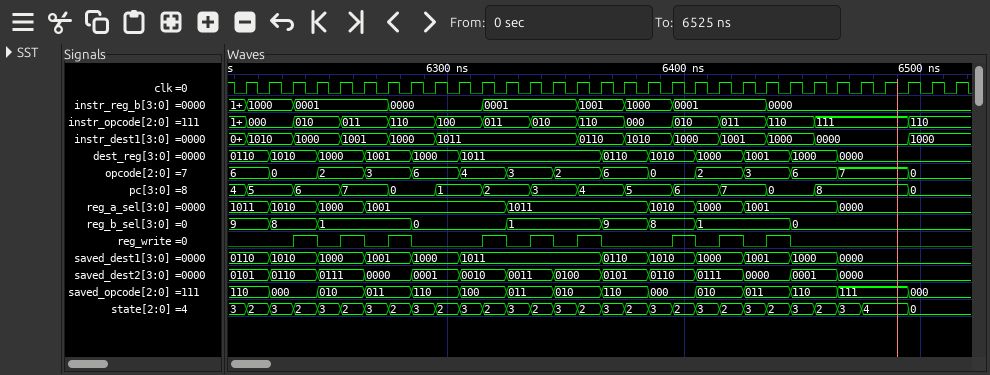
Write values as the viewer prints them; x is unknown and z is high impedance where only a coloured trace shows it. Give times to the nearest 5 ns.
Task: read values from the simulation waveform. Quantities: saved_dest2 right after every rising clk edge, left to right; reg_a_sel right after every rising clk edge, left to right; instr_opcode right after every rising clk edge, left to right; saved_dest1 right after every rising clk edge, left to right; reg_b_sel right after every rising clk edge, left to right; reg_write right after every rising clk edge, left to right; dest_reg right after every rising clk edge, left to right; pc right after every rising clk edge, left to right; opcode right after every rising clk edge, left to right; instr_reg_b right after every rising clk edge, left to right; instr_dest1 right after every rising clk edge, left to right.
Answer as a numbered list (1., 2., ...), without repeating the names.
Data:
1. 0101, 0110, 0110, 0111, 0111, 0000, 0000, 0001, 0001, 0010, 0010, 0011, 0011, 0100, 0100, 0101, 0101, 0110, 0110, 0111, 0111, 0000, 0000, 0001, 0001, 0000, 0000, 0000, 0000, 0000, 0000
2. 1011, 1010, 1010, 1000, 1000, 1001, 1001, 1001, 1001, 1001, 1001, 1011, 1011, 1011, 1011, 1011, 1011, 1010, 1010, 1000, 1000, 1001, 1001, 1001, 1001, 0000, 0000, 0000, 0000, 0000, 0000
3. 000, 000, 010, 010, 011, 011, 110, 110, 100, 100, 011, 011, 010, 010, 110, 110, 000, 000, 010, 010, 011, 011, 110, 110, 111, 111, 111, 111, 110, 110, 110
4. 0110, 1010, 1010, 1000, 1000, 1001, 1001, 1000, 1000, 1011, 1011, 1011, 1011, 1011, 1011, 0110, 0110, 1010, 1010, 1000, 1000, 1001, 1001, 1000, 1000, 0000, 0000, 0000, 0000, 0000, 0000
5. 9, 8, 8, 1, 1, 1, 1, 0, 0, 0, 0, 1, 1, 1, 1, 9, 9, 8, 8, 1, 1, 1, 1, 0, 0, 0, 0, 0, 0, 0, 0
6. 0 0 1 0 1 0 1 0 0 0 1 0 1 0 1 0 0 0 1 0 1 0 1 0 0 0 0 0 0 0 0
7. 0110, 1010, 1010, 1000, 1000, 1001, 1001, 1000, 1000, 1011, 1011, 1011, 1011, 1011, 1011, 0110, 0110, 1010, 1010, 1000, 1000, 1001, 1001, 1000, 1000, 0000, 0000, 0000, 0000, 0000, 0000
8. 5, 5, 6, 6, 7, 7, 0, 0, 1, 1, 2, 2, 3, 3, 4, 4, 5, 5, 6, 6, 7, 7, 0, 0, 8, 8, 8, 8, 0, 0, 0
9. 6, 0, 0, 2, 2, 3, 3, 6, 6, 4, 4, 3, 3, 2, 2, 6, 6, 0, 0, 2, 2, 3, 3, 6, 6, 7, 7, 7, 0, 0, 0
10. 1000, 1000, 0001, 0001, 0001, 0001, 0000, 0000, 0000, 0000, 0001, 0001, 0001, 0001, 1001, 1001, 1000, 1000, 0001, 0001, 0001, 0001, 0000, 0000, 0000, 0000, 0000, 0000, 0000, 0000, 0000
11. 1010, 1010, 1000, 1000, 1001, 1001, 1000, 1000, 1011, 1011, 1011, 1011, 1011, 1011, 0110, 0110, 1010, 1010, 1000, 1000, 1001, 1001, 1000, 1000, 0000, 0000, 0000, 0000, 1000, 1000, 1000
